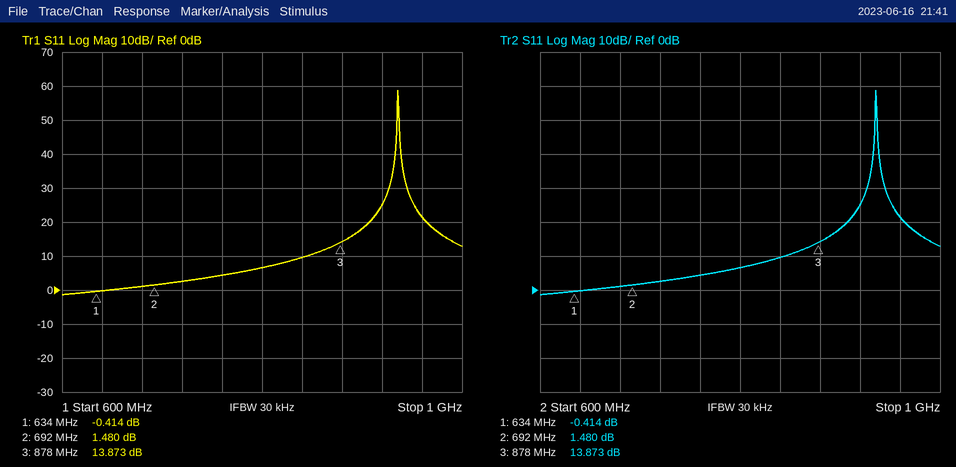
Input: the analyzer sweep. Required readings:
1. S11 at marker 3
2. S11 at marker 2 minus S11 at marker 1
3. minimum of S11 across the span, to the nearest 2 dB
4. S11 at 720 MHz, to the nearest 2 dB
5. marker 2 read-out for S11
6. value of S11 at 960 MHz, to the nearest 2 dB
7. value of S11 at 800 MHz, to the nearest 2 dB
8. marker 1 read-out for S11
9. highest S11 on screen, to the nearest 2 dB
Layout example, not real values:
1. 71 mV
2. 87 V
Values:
1. 13.873 dB
2. 1.894 dB
3. -2 dB
4. 2 dB
5. 1.480 dB
6. 22 dB
7. 6 dB
8. -0.414 dB
9. 58 dB
